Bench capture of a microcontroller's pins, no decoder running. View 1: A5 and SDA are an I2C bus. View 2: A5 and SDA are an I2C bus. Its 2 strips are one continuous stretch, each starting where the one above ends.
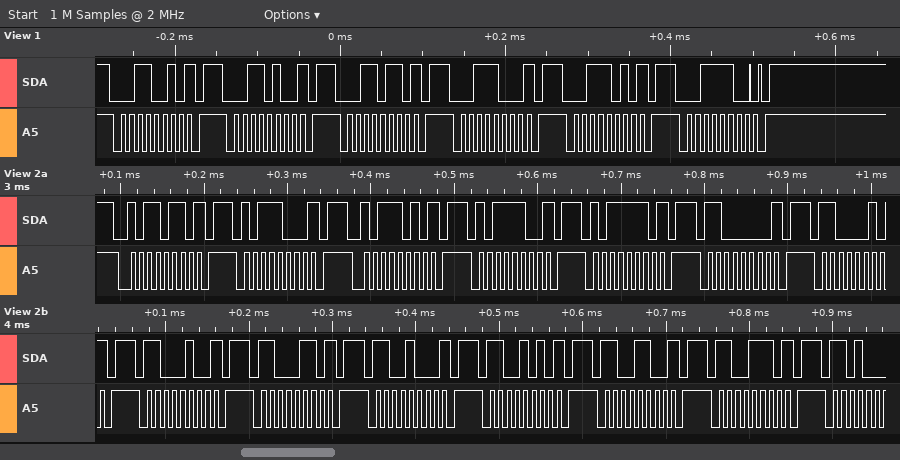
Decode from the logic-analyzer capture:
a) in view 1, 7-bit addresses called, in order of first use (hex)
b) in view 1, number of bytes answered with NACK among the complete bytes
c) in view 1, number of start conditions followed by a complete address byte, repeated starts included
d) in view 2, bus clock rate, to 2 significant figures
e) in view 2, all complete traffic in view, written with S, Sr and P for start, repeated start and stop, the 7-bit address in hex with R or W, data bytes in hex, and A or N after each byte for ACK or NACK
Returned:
0x19 0x1A 0x1B 0x1C 0x1D 0x1E
5
6
100 kHz
S 5BW N P S 5CW N P S 5DW N P S 5EW N P S 5FW N P S 60W N P S 61W N P S 62W N P S 63W N P S 64W N P S 65W N P S 66W N P S 67W N P
